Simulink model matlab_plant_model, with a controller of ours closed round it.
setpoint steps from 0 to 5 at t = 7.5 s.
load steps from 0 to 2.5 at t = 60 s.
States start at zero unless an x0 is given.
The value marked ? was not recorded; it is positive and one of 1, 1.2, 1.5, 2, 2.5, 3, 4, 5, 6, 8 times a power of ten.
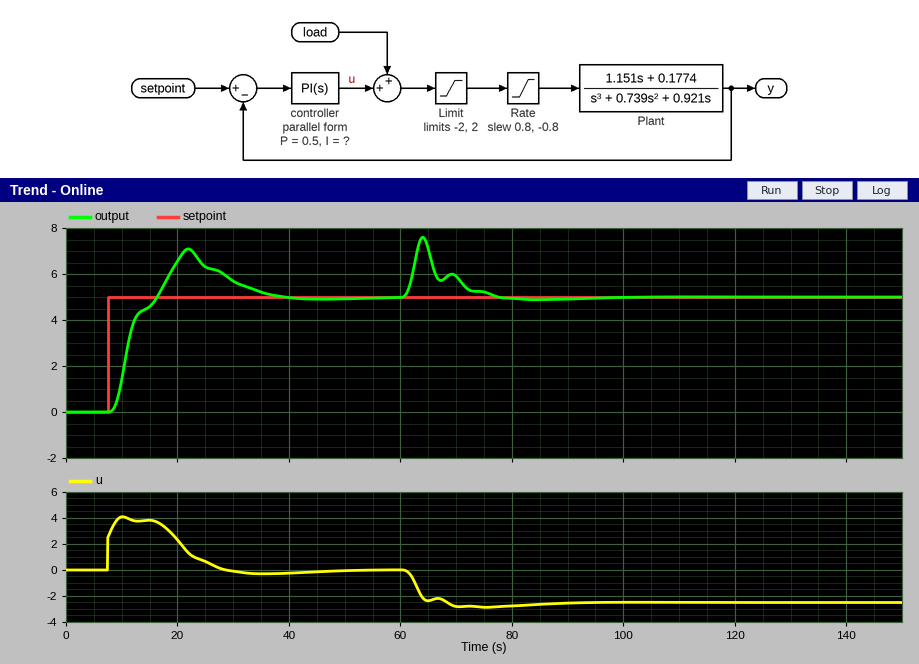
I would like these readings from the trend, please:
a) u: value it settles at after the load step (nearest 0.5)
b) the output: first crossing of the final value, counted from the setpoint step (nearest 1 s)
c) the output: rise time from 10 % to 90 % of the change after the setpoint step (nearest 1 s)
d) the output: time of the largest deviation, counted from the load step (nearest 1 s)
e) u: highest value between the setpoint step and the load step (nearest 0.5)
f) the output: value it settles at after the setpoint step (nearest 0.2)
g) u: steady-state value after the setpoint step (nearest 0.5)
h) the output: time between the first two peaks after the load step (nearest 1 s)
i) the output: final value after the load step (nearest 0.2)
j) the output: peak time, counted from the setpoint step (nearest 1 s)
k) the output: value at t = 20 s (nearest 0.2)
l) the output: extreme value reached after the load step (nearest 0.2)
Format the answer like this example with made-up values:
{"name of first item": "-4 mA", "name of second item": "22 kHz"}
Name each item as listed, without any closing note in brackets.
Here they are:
{"u: value it settles at after the load step": "-2.5", "the output: first crossing of the final value, counted from the setpoint step": "9 s", "the output: rise time from 10 % to 90 % of the change after the setpoint step": "5 s", "the output: time of the largest deviation, counted from the load step": "4 s", "u: highest value between the setpoint step and the load step": "4.0", "the output: value it settles at after the setpoint step": "5.0", "u: steady-state value after the setpoint step": "0.0", "the output: time between the first two peaks after the load step": "5 s", "the output: final value after the load step": "5.0", "the output: peak time, counted from the setpoint step": "14 s", "the output: value at t = 20 s": "6.6", "the output: extreme value reached after the load step": "7.6"}
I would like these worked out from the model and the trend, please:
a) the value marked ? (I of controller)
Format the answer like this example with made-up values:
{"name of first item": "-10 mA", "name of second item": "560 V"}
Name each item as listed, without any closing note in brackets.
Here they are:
{"the value marked ?": "0.2"}
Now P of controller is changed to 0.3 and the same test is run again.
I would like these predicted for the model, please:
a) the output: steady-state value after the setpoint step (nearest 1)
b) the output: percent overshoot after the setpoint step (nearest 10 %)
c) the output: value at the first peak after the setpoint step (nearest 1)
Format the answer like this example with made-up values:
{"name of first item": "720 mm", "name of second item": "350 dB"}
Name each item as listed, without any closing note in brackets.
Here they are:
{"the output: steady-state value after the setpoint step": "5", "the output: percent overshoot after the setpoint step": "50 %", "the output: value at the first peak after the setpoint step": "7"}
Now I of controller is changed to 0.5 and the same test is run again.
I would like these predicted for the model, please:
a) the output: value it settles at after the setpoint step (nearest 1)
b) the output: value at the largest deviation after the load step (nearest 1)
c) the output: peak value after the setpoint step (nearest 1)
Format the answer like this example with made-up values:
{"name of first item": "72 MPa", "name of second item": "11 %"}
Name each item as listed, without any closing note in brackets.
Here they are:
{"the output: value it settles at after the setpoint step": "5", "the output: value at the largest deviation after the load step": "7", "the output: peak value after the setpoint step": "8"}
